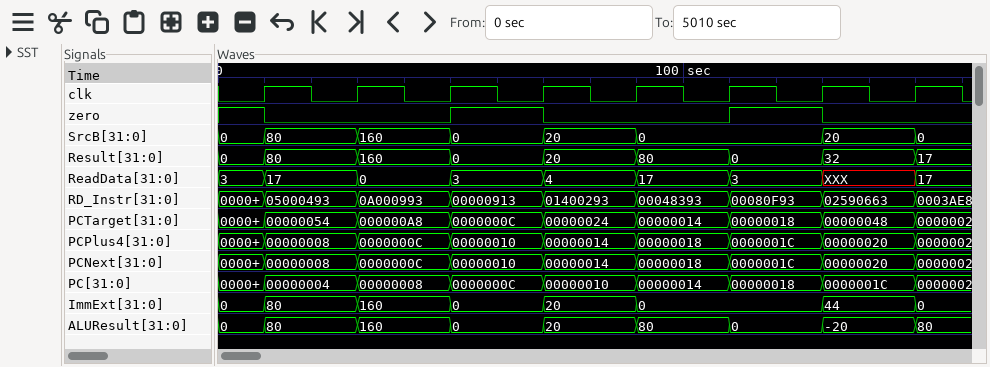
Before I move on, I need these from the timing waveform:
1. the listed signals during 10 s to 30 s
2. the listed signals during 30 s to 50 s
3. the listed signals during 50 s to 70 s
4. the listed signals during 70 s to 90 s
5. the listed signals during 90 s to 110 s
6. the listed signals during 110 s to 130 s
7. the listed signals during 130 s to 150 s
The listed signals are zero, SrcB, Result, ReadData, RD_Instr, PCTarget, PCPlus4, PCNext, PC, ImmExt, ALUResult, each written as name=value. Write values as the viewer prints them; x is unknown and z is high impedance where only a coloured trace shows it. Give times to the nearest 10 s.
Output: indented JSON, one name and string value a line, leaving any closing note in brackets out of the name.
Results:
{
  "the listed signals during 10 s to 30 s": "zero=0, SrcB=80, Result=80, ReadData=17, RD_Instr=05000493, PCTarget=00000054, PCPlus4=00000008, PCNext=00000008, PC=00000004, ImmExt=80, ALUResult=80",
  "the listed signals during 30 s to 50 s": "zero=0, SrcB=160, Result=160, ReadData=0, RD_Instr=0A000993, PCTarget=000000A8, PCPlus4=0000000C, PCNext=0000000C, PC=00000008, ImmExt=160, ALUResult=160",
  "the listed signals during 50 s to 70 s": "zero=1, SrcB=0, Result=0, ReadData=3, RD_Instr=00000913, PCTarget=0000000C, PCPlus4=00000010, PCNext=00000010, PC=0000000C, ImmExt=0, ALUResult=0",
  "the listed signals during 70 s to 90 s": "zero=0, SrcB=20, Result=20, ReadData=4, RD_Instr=01400293, PCTarget=00000024, PCPlus4=00000014, PCNext=00000014, PC=00000010, ImmExt=20, ALUResult=20",
  "the listed signals during 90 s to 110 s": "zero=0, SrcB=0, Result=80, ReadData=17, RD_Instr=00048393, PCTarget=00000014, PCPlus4=00000018, PCNext=00000018, PC=00000014, ImmExt=0, ALUResult=80",
  "the listed signals during 110 s to 130 s": "zero=1, SrcB=0, Result=0, ReadData=3, RD_Instr=00080F93, PCTarget=00000018, PCPlus4=0000001C, PCNext=0000001C, PC=00000018, ImmExt=0, ALUResult=0",
  "the listed signals during 130 s to 150 s": "zero=0, SrcB=20, Result=32, ReadData=XXX, RD_Instr=02590663, PCTarget=00000048, PCPlus4=00000020, PCNext=00000020, PC=0000001C, ImmExt=44, ALUResult=-20"
}
